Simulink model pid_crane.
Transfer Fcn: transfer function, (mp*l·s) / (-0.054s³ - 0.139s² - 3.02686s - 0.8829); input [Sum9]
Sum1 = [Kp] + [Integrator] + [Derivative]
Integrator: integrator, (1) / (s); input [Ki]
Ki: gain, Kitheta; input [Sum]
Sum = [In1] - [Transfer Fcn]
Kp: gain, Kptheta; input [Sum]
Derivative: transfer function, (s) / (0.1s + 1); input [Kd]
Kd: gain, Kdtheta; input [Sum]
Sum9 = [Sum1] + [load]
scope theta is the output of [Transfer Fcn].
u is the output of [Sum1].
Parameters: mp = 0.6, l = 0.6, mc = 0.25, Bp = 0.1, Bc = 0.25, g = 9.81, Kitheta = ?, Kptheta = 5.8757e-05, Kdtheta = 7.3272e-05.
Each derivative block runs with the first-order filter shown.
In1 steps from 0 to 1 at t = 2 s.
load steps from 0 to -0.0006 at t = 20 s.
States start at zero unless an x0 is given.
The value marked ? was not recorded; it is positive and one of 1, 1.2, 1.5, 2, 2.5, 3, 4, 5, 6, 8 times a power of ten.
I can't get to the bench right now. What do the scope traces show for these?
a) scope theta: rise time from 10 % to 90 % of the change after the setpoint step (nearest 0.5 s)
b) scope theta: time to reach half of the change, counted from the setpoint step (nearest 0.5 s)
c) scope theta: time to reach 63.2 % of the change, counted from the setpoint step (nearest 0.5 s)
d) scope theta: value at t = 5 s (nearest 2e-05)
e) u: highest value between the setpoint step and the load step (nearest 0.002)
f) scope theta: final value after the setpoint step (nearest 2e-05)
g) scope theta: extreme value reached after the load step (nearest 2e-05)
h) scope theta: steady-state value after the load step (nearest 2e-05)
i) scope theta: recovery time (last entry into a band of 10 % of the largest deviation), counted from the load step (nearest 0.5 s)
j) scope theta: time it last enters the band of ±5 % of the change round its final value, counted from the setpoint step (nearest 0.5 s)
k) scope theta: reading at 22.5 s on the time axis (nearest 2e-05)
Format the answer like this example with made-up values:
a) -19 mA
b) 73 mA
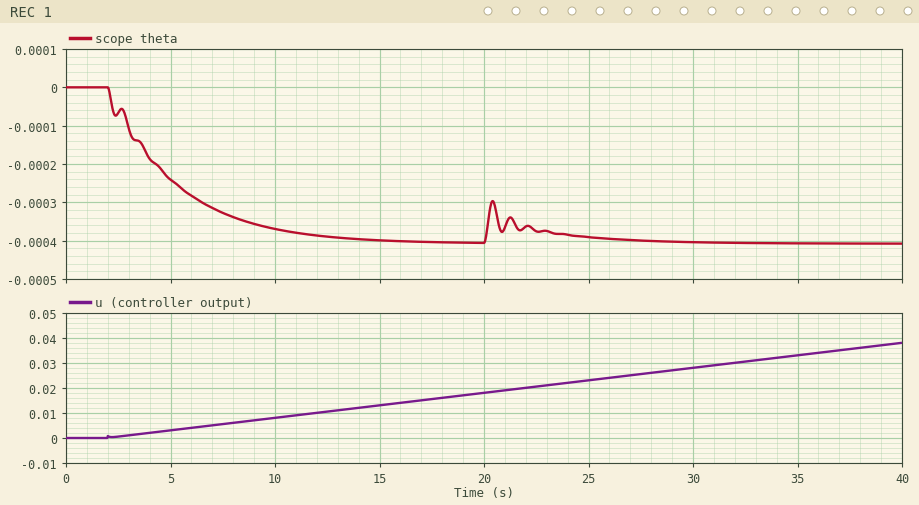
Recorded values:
a) 7.5 s
b) 2.5 s
c) 3.5 s
d) -0.00024
e) 0.018
f) -0.00040
g) -0.00030
h) -0.00040
i) 6.5 s
j) 10.0 s
k) -0.00038
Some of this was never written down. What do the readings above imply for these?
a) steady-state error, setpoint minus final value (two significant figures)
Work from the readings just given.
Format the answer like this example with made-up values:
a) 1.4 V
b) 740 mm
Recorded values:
a) 1.0
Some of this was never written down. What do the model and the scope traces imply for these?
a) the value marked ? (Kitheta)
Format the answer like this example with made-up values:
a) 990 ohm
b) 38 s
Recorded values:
a) 0.001
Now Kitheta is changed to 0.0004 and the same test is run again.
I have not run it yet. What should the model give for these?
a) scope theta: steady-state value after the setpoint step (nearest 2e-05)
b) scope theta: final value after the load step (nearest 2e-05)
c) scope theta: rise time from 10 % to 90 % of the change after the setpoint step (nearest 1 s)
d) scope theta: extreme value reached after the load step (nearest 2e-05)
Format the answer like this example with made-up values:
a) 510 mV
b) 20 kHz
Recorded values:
a) -0.00016
b) -0.00016
c) 8 s
d) -0.00006
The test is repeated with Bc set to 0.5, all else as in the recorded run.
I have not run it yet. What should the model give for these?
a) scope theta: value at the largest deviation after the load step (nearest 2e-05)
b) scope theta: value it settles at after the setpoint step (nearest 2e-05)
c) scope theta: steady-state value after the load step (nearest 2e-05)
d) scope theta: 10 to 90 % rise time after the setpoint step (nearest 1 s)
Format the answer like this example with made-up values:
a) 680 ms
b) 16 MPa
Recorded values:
a) -0.00010
b) -0.00020
c) -0.00020
d) 4 s
